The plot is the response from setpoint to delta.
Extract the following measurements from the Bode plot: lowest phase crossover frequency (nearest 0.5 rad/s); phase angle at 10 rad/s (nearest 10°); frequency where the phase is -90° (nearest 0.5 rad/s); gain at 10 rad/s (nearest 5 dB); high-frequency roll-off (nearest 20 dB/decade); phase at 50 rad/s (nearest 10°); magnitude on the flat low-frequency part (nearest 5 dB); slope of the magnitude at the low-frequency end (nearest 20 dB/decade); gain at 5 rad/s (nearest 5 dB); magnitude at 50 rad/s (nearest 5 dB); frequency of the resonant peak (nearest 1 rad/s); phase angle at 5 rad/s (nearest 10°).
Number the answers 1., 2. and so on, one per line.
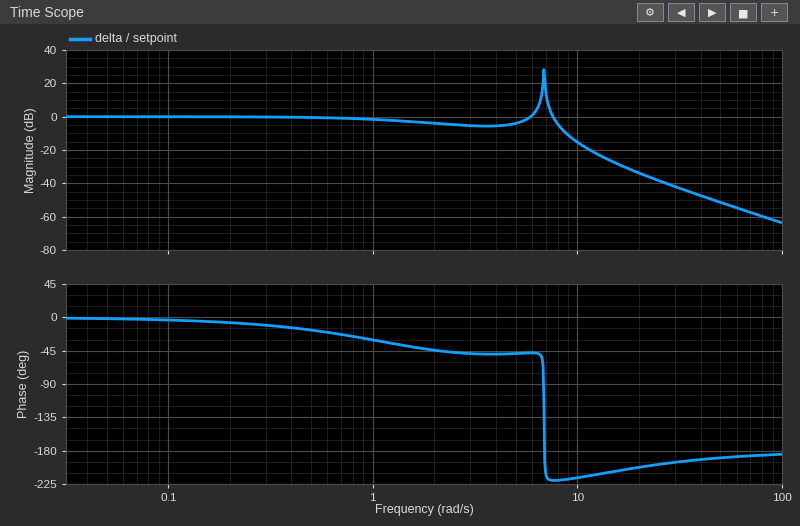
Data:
1. 7.0 rad/s
2. -220°
3. 7.0 rad/s
4. -15 dB
5. -40 dB/decade
6. -190°
7. 0 dB
8. 0 dB/decade
9. -5 dB
10. -50 dB
11. 7 rad/s
12. -50°
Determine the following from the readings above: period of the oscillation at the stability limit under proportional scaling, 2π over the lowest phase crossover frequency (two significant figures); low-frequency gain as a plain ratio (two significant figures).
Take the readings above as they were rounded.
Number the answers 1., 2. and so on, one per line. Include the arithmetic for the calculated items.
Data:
1. 2π / 7 = 0.90 s
2. 10^(0 / 20) = 1.0
